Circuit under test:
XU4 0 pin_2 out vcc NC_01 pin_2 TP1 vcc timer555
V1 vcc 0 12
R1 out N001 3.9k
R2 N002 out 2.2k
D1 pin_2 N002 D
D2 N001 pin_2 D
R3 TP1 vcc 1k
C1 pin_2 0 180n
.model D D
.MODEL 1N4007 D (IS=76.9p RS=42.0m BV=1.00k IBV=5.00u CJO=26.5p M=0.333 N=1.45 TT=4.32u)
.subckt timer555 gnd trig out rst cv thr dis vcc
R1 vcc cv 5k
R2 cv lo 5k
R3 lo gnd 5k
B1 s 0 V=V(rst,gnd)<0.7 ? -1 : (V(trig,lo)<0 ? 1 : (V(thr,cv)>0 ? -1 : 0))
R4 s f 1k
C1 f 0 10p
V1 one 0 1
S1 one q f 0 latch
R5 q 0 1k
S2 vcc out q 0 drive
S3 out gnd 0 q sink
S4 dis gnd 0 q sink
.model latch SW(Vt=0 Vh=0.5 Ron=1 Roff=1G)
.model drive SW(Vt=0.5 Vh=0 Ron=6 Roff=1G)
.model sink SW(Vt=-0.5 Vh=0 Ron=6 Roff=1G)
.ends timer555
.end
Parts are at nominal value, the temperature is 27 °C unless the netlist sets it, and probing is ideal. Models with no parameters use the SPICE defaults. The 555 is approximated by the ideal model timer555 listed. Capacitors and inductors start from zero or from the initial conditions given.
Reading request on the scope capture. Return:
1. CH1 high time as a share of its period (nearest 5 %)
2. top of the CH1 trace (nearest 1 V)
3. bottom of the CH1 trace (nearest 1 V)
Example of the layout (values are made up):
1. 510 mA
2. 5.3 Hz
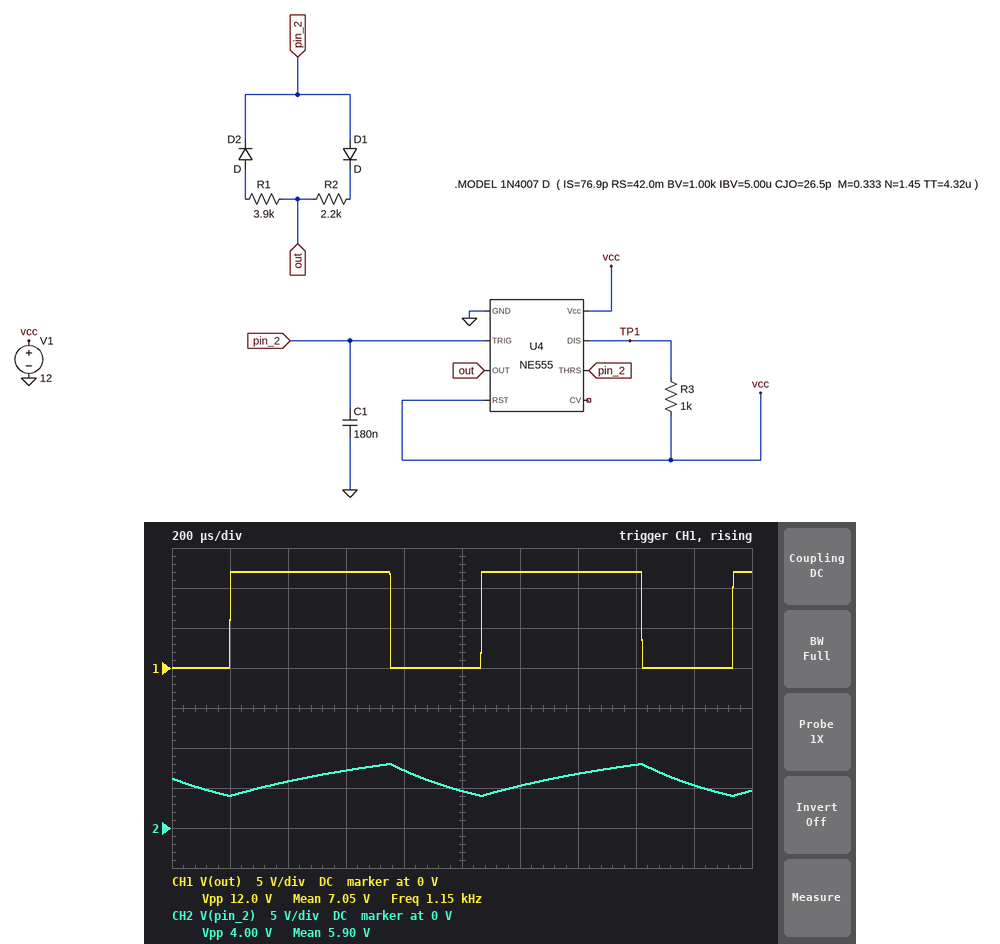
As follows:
1. 65 %
2. 12 V
3. 0 V
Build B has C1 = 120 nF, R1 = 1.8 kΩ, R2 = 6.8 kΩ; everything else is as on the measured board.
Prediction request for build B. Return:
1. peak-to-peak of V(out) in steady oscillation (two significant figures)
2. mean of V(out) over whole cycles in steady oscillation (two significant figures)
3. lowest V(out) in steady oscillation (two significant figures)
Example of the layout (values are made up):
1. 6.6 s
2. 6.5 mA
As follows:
1. 12 V
2. 2.5 V
3. 3.0 mV
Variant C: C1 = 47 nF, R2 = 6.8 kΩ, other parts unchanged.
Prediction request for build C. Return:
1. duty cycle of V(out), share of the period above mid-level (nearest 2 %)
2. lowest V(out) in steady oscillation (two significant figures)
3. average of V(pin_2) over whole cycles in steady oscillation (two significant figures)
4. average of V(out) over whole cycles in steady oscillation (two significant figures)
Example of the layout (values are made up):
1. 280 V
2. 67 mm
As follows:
1. 36 %
2. 3.0 mV
3. 5.9 V
4. 4.4 V
